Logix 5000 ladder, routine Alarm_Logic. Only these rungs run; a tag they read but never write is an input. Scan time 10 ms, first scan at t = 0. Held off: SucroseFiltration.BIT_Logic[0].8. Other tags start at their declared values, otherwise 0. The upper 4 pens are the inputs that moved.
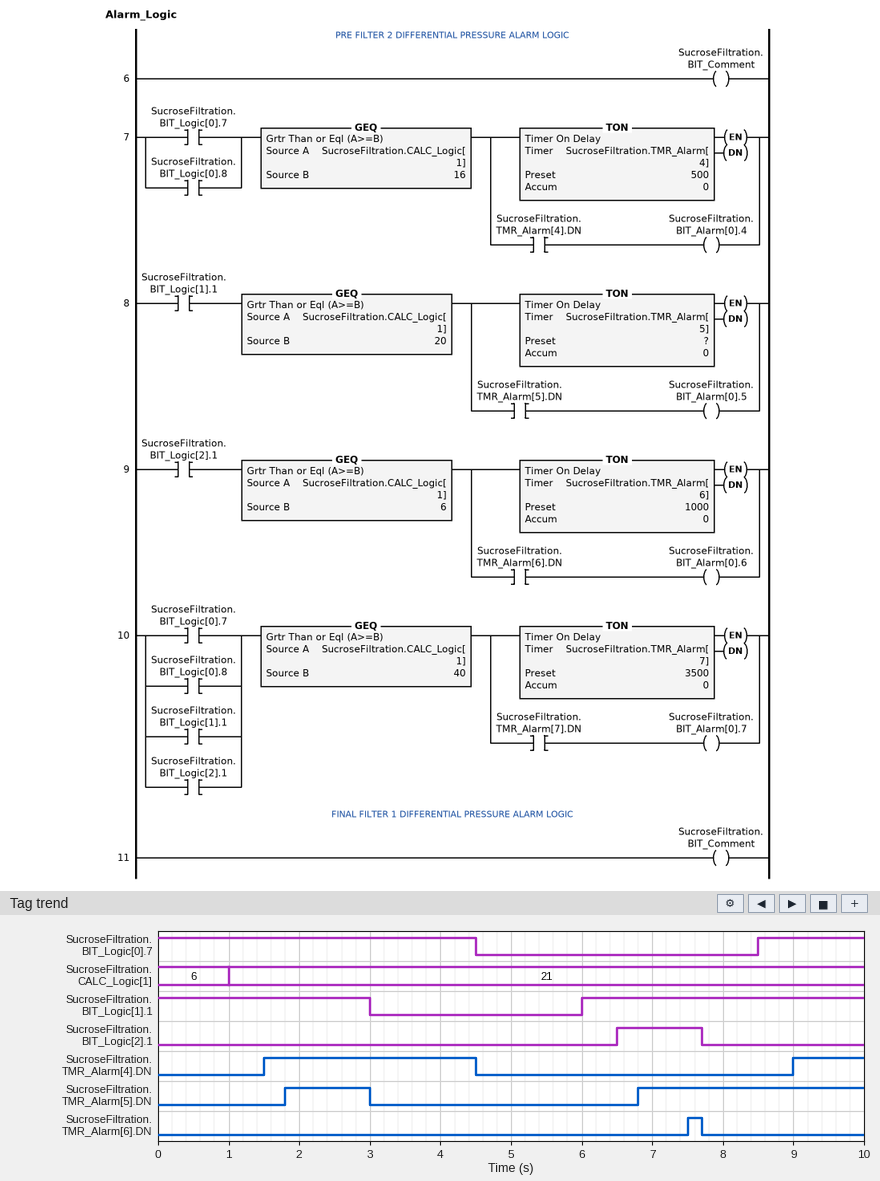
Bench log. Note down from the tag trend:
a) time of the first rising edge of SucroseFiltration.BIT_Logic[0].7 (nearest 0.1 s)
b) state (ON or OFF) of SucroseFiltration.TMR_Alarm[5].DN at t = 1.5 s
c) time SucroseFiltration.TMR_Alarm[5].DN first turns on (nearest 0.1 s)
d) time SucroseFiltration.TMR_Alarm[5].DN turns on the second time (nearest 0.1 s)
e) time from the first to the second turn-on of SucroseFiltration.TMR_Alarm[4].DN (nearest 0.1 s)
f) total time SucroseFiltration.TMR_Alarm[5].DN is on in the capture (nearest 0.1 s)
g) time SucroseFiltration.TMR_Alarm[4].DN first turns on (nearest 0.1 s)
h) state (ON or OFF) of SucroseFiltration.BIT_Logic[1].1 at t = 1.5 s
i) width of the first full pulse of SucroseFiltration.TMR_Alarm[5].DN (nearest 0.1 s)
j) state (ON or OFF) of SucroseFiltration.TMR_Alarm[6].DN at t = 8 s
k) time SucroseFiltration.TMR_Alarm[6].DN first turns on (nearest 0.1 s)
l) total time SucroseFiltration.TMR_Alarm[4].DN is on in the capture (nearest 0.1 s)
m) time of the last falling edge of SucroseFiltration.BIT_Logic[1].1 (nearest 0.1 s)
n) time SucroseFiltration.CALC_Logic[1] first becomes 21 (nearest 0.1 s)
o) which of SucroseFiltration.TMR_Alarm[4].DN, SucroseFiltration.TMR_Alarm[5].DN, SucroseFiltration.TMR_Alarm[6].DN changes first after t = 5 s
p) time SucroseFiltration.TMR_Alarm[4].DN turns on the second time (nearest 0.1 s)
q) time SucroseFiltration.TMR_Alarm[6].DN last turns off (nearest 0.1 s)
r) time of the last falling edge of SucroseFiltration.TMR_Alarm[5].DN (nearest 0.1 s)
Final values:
8.5 s
OFF
1.8 s
6.8 s
7.5 s
4.4 s
1.5 s
ON
1.2 s
OFF
7.5 s
4.0 s
3.0 s
1.0 s
SucroseFiltration.TMR_Alarm[5].DN
9.0 s
7.7 s
3.0 s
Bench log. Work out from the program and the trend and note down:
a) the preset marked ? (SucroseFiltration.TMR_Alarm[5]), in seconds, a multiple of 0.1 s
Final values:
0.8 s
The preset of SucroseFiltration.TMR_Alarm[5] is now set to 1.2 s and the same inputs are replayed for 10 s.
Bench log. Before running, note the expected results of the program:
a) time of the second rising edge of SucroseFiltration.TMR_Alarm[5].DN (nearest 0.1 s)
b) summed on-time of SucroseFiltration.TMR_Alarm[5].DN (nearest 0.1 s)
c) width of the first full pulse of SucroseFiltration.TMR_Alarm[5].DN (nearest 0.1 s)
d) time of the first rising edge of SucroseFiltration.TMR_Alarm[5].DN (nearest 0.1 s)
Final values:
7.2 s
3.6 s
0.8 s
2.2 s
